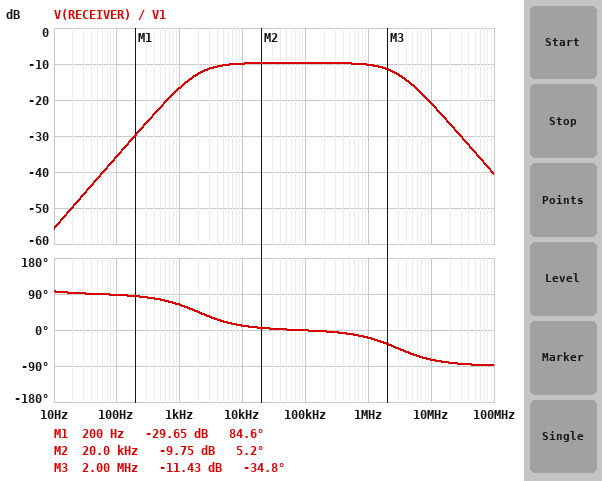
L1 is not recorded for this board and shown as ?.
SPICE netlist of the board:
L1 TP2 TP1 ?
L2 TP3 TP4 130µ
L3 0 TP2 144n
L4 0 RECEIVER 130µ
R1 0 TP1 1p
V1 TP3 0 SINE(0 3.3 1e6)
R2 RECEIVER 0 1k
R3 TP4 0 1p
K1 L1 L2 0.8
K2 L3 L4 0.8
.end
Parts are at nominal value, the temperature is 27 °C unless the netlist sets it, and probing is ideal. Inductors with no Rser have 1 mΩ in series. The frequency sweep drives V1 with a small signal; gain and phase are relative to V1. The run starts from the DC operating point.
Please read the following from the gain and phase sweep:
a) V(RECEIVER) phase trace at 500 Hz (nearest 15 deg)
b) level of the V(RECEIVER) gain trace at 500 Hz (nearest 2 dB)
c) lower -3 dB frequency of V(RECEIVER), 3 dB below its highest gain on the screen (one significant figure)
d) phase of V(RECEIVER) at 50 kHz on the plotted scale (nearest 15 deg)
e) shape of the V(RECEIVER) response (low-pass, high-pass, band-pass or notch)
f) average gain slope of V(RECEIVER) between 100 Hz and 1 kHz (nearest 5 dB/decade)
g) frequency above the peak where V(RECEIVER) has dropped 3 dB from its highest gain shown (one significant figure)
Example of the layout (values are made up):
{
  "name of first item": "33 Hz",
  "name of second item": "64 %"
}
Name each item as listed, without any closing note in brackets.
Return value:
{
  "V(RECEIVER) phase trace at 500 Hz": "75 deg",
  "level of the V(RECEIVER) gain trace at 500 Hz": "-22 dB",
  "lower -3 dB frequency of V(RECEIVER), 3 dB below its highest gain on the screen": "2 kHz",
  "phase of V(RECEIVER) at 50 kHz on the plotted scale": "0 deg",
  "shape of the V(RECEIVER) response": "band-pass",
  "average gain slope of V(RECEIVER) between 100 Hz and 1 kHz": "20 dB/decade",
  "frequency above the peak where V(RECEIVER) has dropped 3 dB from its highest gain shown": "3 MHz"
}
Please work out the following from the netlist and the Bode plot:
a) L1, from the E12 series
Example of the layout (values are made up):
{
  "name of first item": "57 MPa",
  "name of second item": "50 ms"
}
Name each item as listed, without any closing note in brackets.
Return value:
{
  "L1, from the E12 series": "47 nH"
}
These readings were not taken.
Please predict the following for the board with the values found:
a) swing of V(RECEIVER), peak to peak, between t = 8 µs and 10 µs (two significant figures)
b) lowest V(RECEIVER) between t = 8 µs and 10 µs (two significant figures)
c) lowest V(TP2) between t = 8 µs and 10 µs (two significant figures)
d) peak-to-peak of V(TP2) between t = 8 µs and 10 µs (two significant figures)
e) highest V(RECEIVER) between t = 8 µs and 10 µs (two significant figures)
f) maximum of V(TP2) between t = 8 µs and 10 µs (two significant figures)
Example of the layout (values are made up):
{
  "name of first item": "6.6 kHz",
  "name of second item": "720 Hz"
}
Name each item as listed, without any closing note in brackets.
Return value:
{
  "swing of V(RECEIVER), peak to peak, between t = 8 µs and 10 µs": "2.0 V",
  "lowest V(RECEIVER) between t = 8 µs and 10 µs": "-1.0 V",
  "lowest V(TP2) between t = 8 µs and 10 µs": "-44 mV",
  "peak-to-peak of V(TP2) between t = 8 µs and 10 µs": "88 mV",
  "highest V(RECEIVER) between t = 8 µs and 10 µs": "1.0 V",
  "maximum of V(TP2) between t = 8 µs and 10 µs": "44 mV"
}
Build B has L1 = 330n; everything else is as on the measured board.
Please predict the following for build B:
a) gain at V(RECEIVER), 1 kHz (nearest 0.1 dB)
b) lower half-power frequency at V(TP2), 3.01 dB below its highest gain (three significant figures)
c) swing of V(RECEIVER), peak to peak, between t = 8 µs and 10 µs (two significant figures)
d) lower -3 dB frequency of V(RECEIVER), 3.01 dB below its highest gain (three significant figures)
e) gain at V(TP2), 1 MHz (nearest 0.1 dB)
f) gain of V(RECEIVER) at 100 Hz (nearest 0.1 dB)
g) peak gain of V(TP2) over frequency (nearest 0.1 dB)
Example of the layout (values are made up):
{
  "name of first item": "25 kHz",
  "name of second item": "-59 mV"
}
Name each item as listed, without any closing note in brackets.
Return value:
{
  "gain at V(RECEIVER), 1 kHz": "-9.4 dB",
  "lower half-power frequency at V(TP2), 3.01 dB below its highest gain": "1.50 Hz",
  "swing of V(RECEIVER), peak to peak, between t = 8 µs and 10 µs": "3.1 V",
  "lower -3 dB frequency of V(RECEIVER), 3.01 dB below its highest gain": "1.21 kHz",
  "gain at V(TP2), 1 MHz": "-33.8 dB",
  "gain of V(RECEIVER) at 100 Hz": "-27.2 dB",
  "peak gain of V(TP2) over frequency": "-33.1 dB"
}
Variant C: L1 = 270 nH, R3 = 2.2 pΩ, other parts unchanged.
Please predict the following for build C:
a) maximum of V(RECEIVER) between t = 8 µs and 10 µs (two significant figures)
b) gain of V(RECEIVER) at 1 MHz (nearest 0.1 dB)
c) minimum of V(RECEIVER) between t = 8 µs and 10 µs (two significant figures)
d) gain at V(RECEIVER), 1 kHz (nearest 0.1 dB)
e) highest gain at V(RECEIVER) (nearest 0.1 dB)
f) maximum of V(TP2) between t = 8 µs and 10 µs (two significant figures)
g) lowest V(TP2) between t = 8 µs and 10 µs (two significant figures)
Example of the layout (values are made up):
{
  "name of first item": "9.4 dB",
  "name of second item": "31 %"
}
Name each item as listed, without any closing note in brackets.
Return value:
{
  "maximum of V(RECEIVER) between t = 8 µs and 10 µs": "1.5 V",
  "gain of V(RECEIVER) at 1 MHz": "-6.6 dB",
  "minimum of V(RECEIVER) between t = 8 µs and 10 µs": "-1.5 V",
  "gain at V(RECEIVER), 1 kHz": "-10.0 dB",
  "highest gain at V(RECEIVER)": "-5.6 dB",
  "maximum of V(TP2) between t = 8 µs and 10 µs": "67 mV",
  "lowest V(TP2) between t = 8 µs and 10 µs": "-67 mV"
}
